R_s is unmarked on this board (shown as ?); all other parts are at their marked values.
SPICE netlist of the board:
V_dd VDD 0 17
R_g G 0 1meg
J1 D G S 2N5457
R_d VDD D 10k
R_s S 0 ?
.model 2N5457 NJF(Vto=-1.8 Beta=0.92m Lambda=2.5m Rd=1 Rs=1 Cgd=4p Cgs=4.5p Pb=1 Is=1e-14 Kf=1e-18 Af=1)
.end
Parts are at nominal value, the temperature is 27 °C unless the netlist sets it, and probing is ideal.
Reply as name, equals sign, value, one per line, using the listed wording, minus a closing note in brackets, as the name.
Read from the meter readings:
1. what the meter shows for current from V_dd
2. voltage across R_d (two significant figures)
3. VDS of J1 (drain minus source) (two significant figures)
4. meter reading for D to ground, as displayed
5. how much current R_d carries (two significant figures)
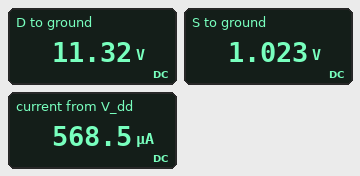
what the meter shows for current from V_dd = 568.5 µA
voltage across R_d = 5.7 V
VDS of J1 (drain minus source) = 10 V
meter reading for D to ground, as displayed = 11.32 V
how much current R_d carries = 570 µA
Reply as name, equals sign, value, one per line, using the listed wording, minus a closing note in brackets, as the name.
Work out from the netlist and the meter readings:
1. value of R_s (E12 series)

value of R_s = 1.8 kΩ
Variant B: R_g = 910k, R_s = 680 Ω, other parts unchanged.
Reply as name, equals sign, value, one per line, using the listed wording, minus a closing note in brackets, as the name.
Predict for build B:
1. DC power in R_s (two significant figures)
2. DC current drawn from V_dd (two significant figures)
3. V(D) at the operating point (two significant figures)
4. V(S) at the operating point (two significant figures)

DC power in R_s = 780 µW
DC current drawn from V_dd = 1.1 mA
V(D) at the operating point = 6.3 V
V(S) at the operating point = 730 mV
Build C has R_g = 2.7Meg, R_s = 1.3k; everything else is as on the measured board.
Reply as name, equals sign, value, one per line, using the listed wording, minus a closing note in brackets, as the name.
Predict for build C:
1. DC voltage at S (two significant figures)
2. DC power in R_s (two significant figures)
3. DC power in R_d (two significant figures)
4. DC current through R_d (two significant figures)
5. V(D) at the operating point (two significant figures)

DC voltage at S = 930 mV
DC power in R_s = 660 µW
DC power in R_d = 5.1 mW
DC current through R_d = 710 µA
V(D) at the operating point = 9.9 V
